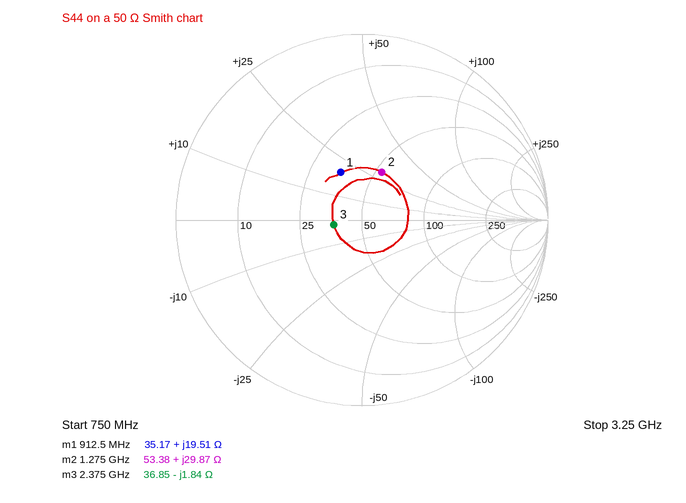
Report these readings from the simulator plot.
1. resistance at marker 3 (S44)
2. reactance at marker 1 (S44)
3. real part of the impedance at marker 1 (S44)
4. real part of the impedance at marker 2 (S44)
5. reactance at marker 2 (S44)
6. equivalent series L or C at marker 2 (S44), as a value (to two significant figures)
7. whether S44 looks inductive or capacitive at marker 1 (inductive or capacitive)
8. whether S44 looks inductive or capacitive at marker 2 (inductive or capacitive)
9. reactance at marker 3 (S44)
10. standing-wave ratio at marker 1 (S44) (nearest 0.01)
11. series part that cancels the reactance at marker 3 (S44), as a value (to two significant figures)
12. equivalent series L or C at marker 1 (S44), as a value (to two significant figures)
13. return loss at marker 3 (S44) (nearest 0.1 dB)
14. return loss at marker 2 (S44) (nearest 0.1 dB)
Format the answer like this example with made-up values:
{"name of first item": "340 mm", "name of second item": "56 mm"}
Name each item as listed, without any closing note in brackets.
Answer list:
{"resistance at marker 3": "36.85 Ω", "reactance at marker 1": "+19.51 Ω", "real part of the impedance at marker 1": "35.17 Ω", "real part of the impedance at marker 2": "53.38 Ω", "reactance at marker 2": "+29.87 Ω", "equivalent series L or C at marker 2 (S44), as a value": "3.7 nH", "whether S44 looks inductive or capacitive at marker 1": "inductive", "whether S44 looks inductive or capacitive at marker 2": "inductive", "reactance at marker 3": "-1.84 Ω", "standing-wave ratio at marker 1 (S44)": "1.78", "series part that cancels the reactance at marker 3 (S44), as a value": "120 pH", "equivalent series L or C at marker 1 (S44), as a value": "3.4 nH", "return loss at marker 3 (S44)": "16.3 dB", "return loss at marker 2 (S44)": "11.1 dB"}
